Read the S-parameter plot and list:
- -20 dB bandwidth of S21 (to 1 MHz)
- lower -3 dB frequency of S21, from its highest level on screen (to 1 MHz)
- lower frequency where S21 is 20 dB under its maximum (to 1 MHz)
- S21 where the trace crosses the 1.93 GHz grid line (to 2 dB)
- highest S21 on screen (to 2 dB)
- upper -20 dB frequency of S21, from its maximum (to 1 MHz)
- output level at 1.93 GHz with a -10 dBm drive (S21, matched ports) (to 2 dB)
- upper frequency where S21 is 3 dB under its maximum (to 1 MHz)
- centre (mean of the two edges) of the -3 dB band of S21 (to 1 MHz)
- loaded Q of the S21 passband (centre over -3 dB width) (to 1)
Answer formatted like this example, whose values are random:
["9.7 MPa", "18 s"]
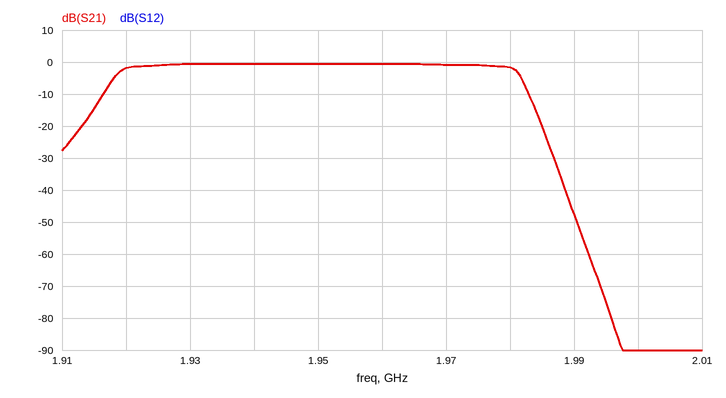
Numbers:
["72 MHz", "1.919 GHz", "1.913 GHz", "0 dB", "0 dB", "1.985 GHz", "-10 dBm", "1.981 GHz", "1.950 GHz", "31"]
